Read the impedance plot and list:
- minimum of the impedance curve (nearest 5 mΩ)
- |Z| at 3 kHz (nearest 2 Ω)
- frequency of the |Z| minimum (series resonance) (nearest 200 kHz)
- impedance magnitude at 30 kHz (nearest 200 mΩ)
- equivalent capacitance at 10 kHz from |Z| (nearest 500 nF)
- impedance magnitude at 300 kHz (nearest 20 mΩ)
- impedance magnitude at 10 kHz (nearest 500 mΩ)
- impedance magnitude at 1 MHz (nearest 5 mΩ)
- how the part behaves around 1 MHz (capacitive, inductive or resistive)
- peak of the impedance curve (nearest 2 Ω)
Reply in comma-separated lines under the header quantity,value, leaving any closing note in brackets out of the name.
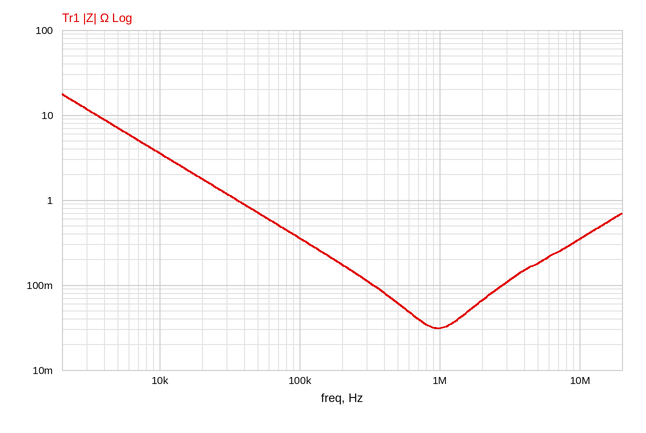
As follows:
quantity,value
minimum of the impedance curve,30 mΩ
|Z| at 3 kHz,12 Ω
frequency of the |Z| minimum (series resonance),1.0 MHz
impedance magnitude at 30 kHz,1.2 Ω
equivalent capacitance at 10 kHz from |Z|,4.5 µF
impedance magnitude at 300 kHz,120 mΩ
impedance magnitude at 10 kHz,3.5 Ω
impedance magnitude at 1 MHz,30 mΩ
how the part behaves around 1 MHz,resistive
peak of the impedance curve,18 Ω
